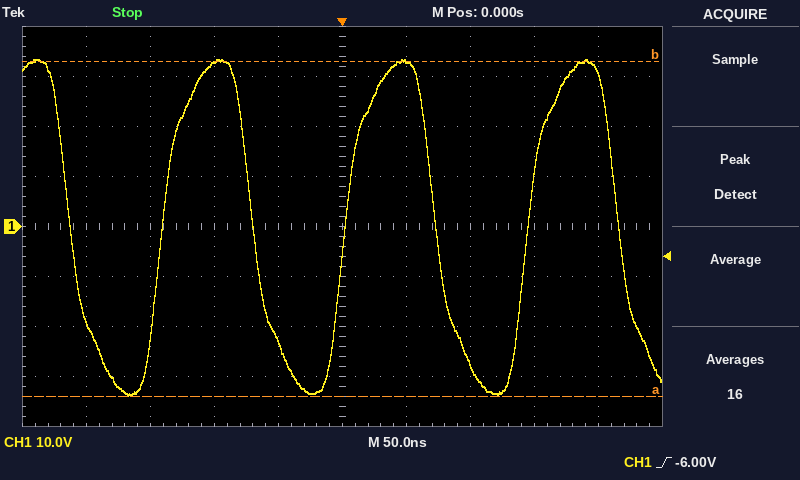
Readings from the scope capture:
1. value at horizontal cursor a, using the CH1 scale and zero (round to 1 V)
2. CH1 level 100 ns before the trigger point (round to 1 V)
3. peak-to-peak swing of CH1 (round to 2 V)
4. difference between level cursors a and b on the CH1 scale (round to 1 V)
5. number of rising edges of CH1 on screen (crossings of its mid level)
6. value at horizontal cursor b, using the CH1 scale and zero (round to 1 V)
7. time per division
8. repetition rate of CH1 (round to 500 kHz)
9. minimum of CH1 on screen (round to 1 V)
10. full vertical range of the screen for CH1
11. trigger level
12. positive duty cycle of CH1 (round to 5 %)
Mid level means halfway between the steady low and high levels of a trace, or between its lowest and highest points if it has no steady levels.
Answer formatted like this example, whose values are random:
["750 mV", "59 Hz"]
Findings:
["-34 V", "33 V", "68 V", "67 V", "3", "33 V", "50 ns", "7.0 MHz", "-34 V", "80 V", "-6.00 V", "50 %"]
